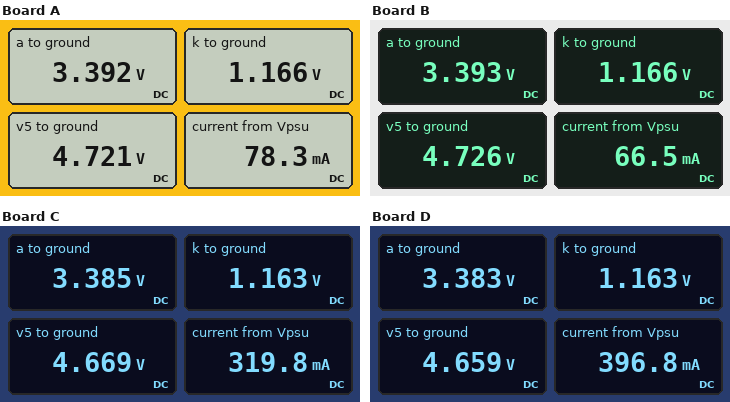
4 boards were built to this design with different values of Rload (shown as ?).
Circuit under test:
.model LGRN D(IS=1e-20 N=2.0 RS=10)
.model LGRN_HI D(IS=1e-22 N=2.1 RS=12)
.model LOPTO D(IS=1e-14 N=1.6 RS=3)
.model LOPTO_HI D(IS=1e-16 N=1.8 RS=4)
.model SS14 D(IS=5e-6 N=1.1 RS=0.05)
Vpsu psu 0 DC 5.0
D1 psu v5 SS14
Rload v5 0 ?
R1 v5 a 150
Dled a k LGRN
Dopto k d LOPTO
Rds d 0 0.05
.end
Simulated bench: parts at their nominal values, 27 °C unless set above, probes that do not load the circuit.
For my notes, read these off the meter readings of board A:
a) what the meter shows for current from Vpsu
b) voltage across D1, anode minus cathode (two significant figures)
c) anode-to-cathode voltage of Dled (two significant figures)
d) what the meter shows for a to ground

78.3 mA
280 mV
2.2 V
3.392 V
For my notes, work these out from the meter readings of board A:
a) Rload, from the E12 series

68 Ω
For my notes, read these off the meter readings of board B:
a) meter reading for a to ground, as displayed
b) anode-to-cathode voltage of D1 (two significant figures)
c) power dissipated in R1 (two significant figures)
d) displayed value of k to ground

3.393 V
270 mV
12 mW
1.166 V
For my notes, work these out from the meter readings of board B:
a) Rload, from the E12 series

82 Ω
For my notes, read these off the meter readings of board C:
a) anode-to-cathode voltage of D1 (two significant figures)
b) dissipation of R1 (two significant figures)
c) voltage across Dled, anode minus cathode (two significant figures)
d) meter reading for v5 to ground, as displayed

330 mV
11 mW
2.2 V
4.669 V
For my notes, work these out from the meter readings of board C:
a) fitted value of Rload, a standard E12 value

15 Ω
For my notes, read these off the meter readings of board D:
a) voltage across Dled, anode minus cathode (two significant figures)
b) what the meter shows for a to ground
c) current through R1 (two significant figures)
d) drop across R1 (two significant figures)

2.2 V
3.383 V
8.5 mA
1.3 V
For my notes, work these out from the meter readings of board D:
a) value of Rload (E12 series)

12 Ω
